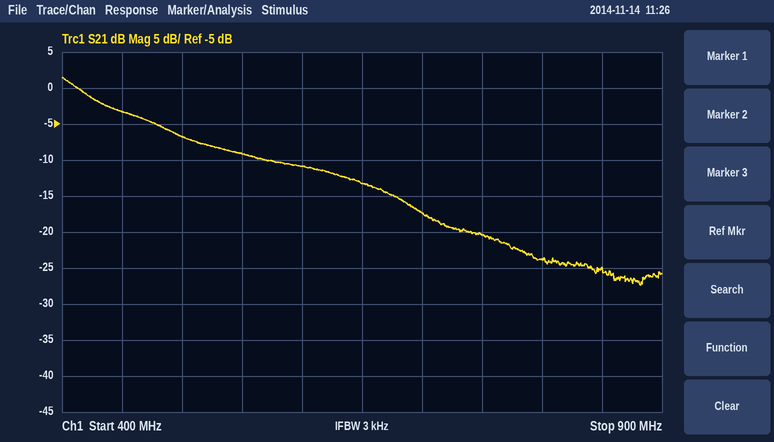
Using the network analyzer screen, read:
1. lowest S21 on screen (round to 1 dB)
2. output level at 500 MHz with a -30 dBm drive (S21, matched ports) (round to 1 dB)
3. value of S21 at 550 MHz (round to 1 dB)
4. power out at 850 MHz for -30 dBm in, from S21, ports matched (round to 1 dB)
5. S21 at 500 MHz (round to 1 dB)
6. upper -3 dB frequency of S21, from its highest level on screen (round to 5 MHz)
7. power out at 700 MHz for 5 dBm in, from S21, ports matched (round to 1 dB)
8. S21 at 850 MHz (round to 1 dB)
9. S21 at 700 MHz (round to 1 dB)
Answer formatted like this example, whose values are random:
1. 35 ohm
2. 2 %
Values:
1. -27 dB
2. -37 dBm
3. -9 dB
4. -55 dBm
5. -7 dB
6. 425 MHz
7. -12 dBm
8. -25 dB
9. -17 dB
